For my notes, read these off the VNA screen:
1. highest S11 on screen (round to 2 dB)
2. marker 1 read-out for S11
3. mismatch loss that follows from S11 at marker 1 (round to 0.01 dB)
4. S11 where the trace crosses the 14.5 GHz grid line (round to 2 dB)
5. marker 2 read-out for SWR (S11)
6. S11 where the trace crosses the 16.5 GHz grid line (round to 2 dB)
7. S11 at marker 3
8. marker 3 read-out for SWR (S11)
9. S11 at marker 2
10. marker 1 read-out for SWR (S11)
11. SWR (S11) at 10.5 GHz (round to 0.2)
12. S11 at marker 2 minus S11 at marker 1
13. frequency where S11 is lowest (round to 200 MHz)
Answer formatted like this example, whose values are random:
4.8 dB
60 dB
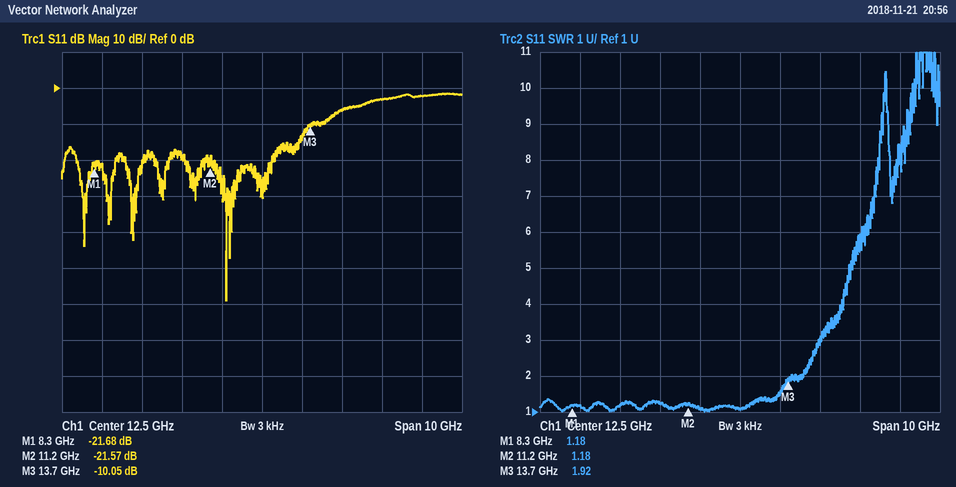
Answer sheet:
-2 dB
-21.68 dB
0.03 dB
-6 dB
1.18
-2 dB
-10.05 dB
1.92
-21.57 dB
1.18
1.2
0.11 dB
11.6 GHz
